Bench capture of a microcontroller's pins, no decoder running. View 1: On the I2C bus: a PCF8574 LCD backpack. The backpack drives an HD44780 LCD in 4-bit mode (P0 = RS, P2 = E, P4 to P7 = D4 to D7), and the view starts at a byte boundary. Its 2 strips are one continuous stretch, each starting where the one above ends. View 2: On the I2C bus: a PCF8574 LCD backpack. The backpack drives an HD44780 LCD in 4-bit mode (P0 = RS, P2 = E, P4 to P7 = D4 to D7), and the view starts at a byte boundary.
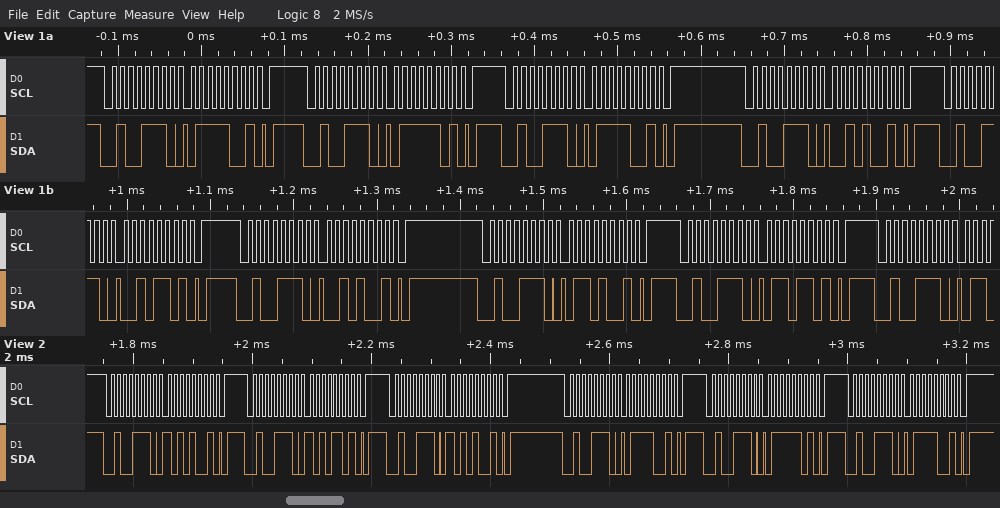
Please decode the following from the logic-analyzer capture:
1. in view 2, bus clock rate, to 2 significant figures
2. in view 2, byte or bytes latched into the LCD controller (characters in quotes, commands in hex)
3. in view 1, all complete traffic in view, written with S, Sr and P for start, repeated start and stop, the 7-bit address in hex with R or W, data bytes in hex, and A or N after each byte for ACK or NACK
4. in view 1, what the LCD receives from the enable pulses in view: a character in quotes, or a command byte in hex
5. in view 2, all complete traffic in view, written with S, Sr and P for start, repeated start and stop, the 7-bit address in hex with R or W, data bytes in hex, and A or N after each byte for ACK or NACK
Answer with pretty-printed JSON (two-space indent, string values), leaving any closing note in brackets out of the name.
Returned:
{
  "in view 2, bus clock rate, to 2 significant figures": "100 kHz",
  "in view 2, byte or bytes latched into the LCD controller": "data 0xA7",
  "in view 1, all complete traffic in view, written with S, Sr and P for start, repeated start and stop, the 7-bit address in hex with R or W, data bytes in hex, and A or N after each byte for ACK or NACK": "S 27W A 79 A P S 27W A 7D A P S 27W A 79 A P S 27W A 29 A P S 27W A 2D A P S 27W A 29 A P S 27W A 69 A P S 27W A 6D A P S 27W A",
  "in view 1, what the LCD receives from the enable pulses in view: a character in quotes, or a command byte in hex": "'r'",
  "in view 2, all complete traffic in view, written with S, Sr and P for start, repeated start and stop, the 7-bit address in hex with R or W, data bytes in hex, and A or N after each byte for ACK or NACK": "S 27W A A9 A P S 27W A AD A P S 27W A A9 A P S 27W A 79 A P S 27W A 7D A P S 27W A 79 A P"
}
